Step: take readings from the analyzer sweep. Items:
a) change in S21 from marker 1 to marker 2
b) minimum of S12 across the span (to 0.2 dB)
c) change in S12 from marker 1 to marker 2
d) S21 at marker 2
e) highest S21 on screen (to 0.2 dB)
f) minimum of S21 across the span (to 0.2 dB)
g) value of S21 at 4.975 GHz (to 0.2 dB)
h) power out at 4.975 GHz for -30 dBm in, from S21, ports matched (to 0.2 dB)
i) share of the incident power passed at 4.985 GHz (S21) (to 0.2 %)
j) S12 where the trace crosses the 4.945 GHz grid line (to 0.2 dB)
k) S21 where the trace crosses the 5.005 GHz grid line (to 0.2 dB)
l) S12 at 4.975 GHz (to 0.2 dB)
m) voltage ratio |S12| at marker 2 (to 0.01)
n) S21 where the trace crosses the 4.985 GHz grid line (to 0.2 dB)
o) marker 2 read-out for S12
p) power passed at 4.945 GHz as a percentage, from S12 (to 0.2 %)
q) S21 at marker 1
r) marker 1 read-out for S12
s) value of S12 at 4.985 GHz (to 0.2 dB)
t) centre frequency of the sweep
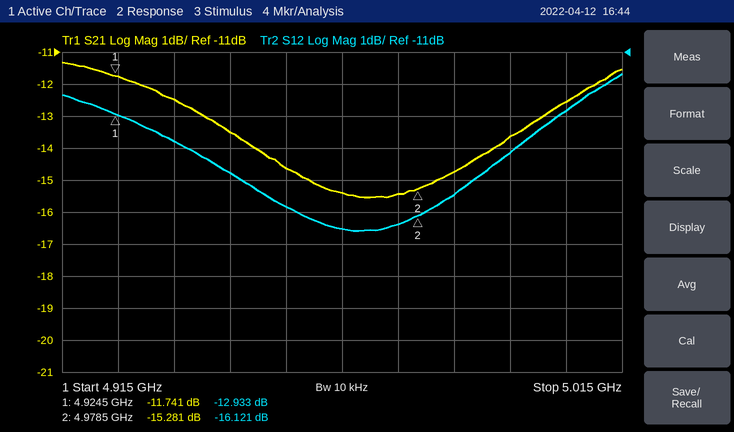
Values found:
-3.540 dB
-16.6 dB
-3.188 dB
-15.281 dB
-11.4 dB
-15.6 dB
-15.4 dB
-45.4 dBm
3.4 %
-14.8 dB
-12.6 dB
-16.4 dB
0.16
-14.8 dB
-16.121 dB
3.4 %
-11.741 dB
-12.933 dB
-15.4 dB
4.965 GHz
